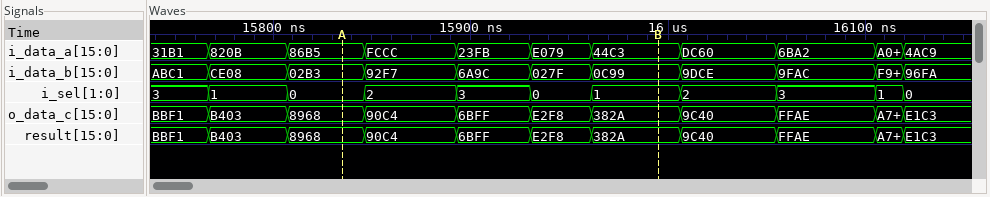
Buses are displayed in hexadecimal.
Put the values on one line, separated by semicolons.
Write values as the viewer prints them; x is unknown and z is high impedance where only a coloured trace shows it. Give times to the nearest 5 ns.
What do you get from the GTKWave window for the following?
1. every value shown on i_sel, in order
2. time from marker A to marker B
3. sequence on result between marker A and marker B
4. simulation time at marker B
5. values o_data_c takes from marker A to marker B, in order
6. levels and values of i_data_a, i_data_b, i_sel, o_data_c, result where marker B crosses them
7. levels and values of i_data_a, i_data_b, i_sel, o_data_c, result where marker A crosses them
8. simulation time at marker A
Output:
3, 1, 0, 2, 3, 0, 1, 2, 3, 1, 0; 160 ns; 8968, 90C4, 6BFF, E2F8, 382A; 15995 ns; 8968, 90C4, 6BFF, E2F8, 382A; i_data_a=44C3, i_data_b=0C99, i_sel=1, o_data_c=382A, result=382A; i_data_a=86B5, i_data_b=02B3, i_sel=0, o_data_c=8968, result=8968; 15835 ns
